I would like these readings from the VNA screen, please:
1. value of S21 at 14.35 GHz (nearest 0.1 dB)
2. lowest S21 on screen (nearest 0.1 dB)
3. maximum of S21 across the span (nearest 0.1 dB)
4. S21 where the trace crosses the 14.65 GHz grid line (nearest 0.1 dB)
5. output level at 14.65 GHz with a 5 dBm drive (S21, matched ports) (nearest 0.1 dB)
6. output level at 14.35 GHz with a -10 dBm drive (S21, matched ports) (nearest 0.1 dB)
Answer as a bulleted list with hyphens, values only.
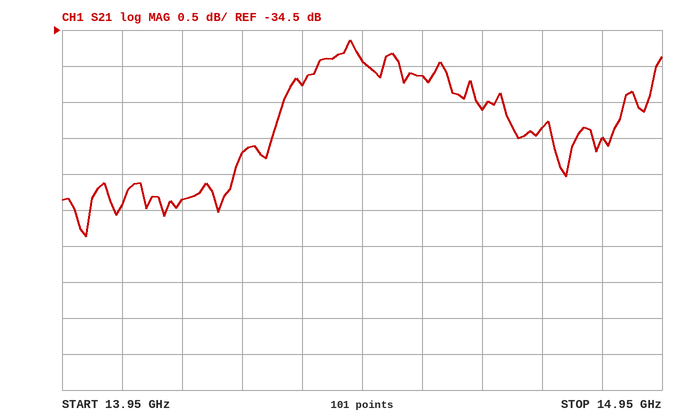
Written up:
- -35.3 dB
- -37.4 dB
- -34.6 dB
- -35.6 dB
- -30.6 dBm
- -45.3 dBm
